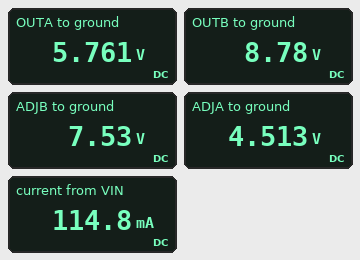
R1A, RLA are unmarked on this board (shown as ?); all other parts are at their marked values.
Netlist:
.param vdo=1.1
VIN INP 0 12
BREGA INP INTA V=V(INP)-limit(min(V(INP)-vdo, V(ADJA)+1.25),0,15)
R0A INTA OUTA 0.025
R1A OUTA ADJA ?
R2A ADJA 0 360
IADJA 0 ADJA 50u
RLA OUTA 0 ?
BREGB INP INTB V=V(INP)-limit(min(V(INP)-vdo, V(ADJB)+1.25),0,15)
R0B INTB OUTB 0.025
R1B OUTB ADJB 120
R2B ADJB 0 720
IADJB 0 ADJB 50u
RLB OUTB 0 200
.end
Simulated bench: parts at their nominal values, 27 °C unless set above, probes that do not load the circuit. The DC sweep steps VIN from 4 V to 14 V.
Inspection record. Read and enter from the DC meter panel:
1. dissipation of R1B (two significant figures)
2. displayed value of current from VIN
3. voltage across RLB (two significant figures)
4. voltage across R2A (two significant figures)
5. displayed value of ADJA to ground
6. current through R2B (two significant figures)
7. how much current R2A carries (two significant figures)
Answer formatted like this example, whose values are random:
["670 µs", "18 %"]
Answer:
["13 mW", "114.8 mA", "8.8 V", "4.5 V", "4.513 V", "10 mA", "13 mA"]
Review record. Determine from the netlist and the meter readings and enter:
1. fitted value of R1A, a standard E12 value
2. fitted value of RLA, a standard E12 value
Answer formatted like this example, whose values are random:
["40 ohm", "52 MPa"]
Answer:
["100 Ω", "120 Ω"]
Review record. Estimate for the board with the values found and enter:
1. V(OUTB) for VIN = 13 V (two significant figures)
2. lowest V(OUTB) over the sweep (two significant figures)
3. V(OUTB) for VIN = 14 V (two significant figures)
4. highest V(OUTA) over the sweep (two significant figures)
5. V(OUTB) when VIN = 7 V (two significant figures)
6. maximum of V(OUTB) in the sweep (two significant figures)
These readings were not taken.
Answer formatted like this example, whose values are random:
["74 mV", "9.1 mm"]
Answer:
["8.8 V", "2.9 V", "8.8 V", "5.8 V", "5.9 V", "8.8 V"]
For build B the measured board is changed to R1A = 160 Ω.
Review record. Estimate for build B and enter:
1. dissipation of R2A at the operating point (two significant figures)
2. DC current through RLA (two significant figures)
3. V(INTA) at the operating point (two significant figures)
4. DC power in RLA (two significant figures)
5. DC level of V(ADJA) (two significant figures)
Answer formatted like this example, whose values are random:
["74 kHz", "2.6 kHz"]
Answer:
["22 mW", "34 mA", "4.1 V", "140 mW", "2.8 V"]
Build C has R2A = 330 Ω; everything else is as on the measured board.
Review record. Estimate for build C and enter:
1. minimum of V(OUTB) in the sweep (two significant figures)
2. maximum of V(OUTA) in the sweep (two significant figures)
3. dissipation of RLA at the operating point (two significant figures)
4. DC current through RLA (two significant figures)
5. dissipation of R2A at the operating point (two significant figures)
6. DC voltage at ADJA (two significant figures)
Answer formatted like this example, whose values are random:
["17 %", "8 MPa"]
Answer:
["2.9 V", "5.4 V", "240 mW", "45 mA", "52 mW", "4.1 V"]
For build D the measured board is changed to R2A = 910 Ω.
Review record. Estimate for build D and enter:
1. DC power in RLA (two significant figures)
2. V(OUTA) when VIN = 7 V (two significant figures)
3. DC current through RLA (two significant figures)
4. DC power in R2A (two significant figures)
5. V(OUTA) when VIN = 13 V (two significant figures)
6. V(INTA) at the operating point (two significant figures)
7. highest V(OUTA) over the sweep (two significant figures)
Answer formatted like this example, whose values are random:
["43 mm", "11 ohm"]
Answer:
["990 mW", "5.9 V", "91 mA", "110 mW", "12 V", "11 V", "13 V"]
